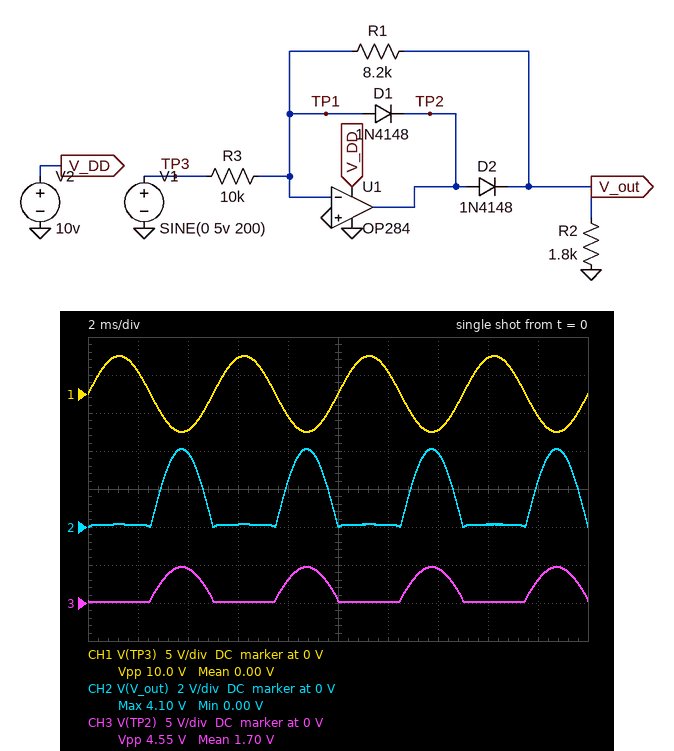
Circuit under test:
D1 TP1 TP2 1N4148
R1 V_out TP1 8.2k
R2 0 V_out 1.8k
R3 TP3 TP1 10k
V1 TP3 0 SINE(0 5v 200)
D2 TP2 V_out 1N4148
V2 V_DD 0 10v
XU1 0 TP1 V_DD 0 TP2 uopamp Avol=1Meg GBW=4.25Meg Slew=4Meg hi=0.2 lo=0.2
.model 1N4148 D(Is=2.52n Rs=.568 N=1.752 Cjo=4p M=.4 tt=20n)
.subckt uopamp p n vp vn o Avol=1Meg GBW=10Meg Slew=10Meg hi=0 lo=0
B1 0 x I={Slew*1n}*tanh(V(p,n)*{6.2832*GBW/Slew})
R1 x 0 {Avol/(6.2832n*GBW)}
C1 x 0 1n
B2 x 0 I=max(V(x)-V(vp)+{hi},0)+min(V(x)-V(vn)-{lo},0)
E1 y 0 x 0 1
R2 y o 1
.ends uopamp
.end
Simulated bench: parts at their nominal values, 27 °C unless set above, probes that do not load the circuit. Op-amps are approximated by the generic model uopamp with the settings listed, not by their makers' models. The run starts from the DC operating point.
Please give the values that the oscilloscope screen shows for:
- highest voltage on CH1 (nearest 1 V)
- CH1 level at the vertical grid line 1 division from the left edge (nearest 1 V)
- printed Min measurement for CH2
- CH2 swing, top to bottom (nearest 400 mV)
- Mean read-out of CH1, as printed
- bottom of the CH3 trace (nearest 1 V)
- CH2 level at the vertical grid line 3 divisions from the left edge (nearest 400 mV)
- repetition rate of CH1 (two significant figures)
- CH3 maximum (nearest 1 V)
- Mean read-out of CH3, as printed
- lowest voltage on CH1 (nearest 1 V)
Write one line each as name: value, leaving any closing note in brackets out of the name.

highest voltage on CH1: 5 V
CH1 level at the vertical grid line 1 division from the left edge: 3 V
printed Min measurement for CH2: 0.00 V
CH2 swing, top to bottom: 4.0 V
Mean read-out of CH1, as printed: 0.00 V
bottom of the CH3 trace: 0 V
CH2 level at the vertical grid line 3 divisions from the left edge: 0 V
repetition rate of CH1: 200 Hz
CH3 maximum: 5 V
Mean read-out of CH3, as printed: 1.70 V
lowest voltage on CH1: -5 V
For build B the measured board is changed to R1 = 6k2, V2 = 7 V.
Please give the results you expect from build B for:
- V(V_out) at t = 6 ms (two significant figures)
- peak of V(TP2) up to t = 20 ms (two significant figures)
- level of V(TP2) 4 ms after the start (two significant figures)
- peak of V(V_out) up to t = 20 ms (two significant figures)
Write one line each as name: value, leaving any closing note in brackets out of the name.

V(V_out) at t = 6 ms: 160 mV
peak of V(TP2) up to t = 20 ms: 3.7 V
level of V(TP2) 4 ms after the start: 3.6 V
peak of V(V_out) up to t = 20 ms: 3.1 V
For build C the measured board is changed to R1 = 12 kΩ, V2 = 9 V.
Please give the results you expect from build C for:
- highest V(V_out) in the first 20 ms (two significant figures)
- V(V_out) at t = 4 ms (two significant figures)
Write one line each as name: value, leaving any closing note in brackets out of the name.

highest V(V_out) in the first 20 ms: 6.0 V
V(V_out) at t = 4 ms: 5.7 V
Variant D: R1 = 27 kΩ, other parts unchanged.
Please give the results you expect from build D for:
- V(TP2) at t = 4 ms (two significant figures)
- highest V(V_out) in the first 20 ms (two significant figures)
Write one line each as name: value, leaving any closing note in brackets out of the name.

V(TP2) at t = 4 ms: 9.8 V
highest V(V_out) in the first 20 ms: 9.1 V
